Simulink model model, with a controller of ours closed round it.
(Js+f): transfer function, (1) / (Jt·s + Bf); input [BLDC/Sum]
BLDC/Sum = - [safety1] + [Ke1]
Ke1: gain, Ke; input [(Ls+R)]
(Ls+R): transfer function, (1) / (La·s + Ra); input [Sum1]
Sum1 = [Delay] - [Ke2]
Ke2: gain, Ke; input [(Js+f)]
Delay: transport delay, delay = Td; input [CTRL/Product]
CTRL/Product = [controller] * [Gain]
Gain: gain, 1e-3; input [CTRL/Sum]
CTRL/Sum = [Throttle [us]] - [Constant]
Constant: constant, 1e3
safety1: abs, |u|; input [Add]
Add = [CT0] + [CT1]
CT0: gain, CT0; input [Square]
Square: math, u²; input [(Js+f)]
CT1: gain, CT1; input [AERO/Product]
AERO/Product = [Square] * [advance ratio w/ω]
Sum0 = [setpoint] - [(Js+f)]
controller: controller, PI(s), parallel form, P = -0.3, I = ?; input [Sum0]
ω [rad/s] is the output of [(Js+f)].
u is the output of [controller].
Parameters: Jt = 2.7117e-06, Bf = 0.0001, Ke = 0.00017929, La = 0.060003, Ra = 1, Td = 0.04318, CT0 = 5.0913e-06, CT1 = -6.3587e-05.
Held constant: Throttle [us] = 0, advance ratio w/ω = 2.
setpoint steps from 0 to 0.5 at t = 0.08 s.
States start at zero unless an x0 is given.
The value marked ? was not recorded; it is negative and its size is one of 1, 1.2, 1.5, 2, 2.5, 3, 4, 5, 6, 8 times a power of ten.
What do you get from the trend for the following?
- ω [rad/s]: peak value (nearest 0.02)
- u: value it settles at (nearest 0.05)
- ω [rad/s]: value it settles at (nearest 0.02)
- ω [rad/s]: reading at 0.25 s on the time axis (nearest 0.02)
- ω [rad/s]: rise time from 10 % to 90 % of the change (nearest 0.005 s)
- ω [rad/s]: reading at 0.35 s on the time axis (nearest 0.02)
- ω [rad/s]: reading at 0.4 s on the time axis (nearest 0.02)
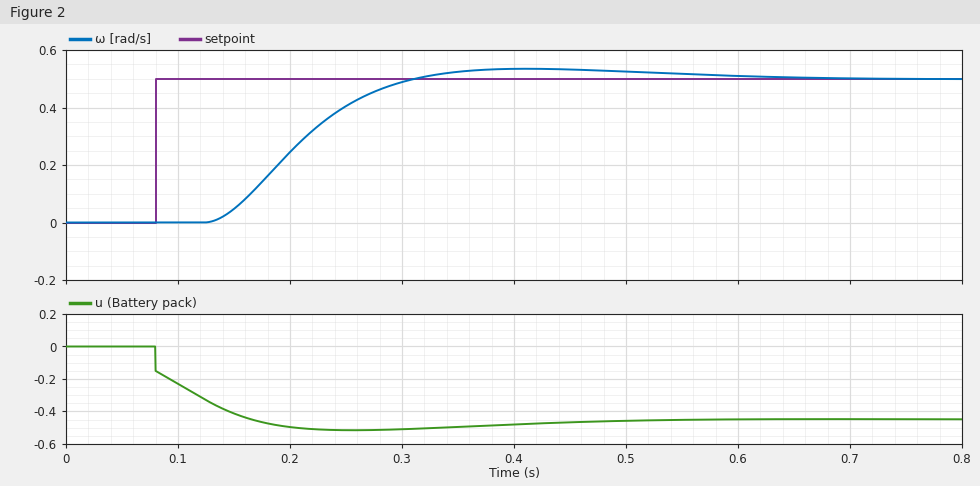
0.54
-0.45
0.50
0.40
0.120 s
0.52
0.54
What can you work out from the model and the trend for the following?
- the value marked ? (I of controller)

-8
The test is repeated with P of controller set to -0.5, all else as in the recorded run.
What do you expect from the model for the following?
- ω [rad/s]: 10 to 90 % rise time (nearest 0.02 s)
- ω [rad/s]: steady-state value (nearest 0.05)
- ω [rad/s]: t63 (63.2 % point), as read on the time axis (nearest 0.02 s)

0.10 s
0.50
0.20 s
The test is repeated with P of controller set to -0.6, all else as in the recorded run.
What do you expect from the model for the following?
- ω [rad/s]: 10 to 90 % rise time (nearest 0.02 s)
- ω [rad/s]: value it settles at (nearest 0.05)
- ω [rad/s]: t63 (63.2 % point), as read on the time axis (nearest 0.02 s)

0.10 s
0.50
0.20 s
